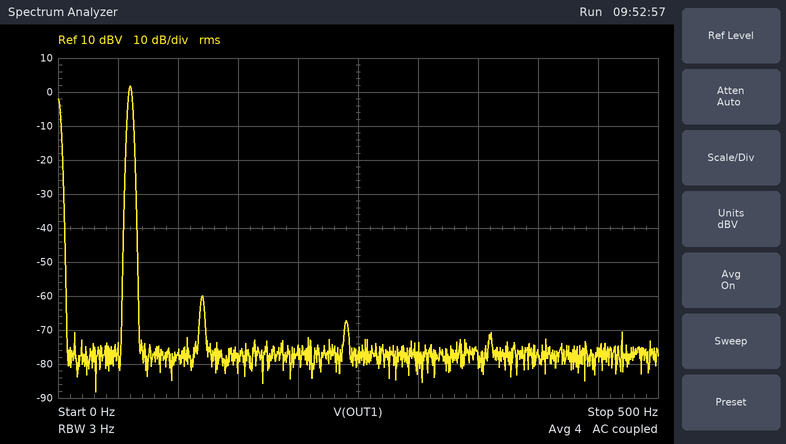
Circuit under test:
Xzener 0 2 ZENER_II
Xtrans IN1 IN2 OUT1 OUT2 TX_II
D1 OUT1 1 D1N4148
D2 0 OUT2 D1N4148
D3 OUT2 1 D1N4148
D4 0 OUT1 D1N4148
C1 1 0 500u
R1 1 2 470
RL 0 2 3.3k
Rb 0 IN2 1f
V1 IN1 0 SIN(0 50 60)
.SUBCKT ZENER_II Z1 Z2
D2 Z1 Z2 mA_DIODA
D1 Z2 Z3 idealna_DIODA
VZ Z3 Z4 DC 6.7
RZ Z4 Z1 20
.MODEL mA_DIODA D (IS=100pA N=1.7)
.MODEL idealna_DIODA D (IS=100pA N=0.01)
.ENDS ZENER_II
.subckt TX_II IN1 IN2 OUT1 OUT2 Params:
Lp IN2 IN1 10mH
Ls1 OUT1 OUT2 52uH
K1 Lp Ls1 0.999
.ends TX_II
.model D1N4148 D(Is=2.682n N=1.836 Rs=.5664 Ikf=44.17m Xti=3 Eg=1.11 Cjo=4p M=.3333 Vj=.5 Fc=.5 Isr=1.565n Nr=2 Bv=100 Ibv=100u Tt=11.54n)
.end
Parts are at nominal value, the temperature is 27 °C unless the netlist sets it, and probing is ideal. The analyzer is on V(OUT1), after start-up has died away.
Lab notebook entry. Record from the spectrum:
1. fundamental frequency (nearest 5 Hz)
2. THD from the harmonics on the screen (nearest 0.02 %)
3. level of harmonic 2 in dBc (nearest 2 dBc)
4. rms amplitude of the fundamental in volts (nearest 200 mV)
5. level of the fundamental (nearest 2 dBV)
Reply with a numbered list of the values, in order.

1. 60 Hz
2. 0.08 %
3. -62 dBc
4. 1.2 V
5. 2 dBV
